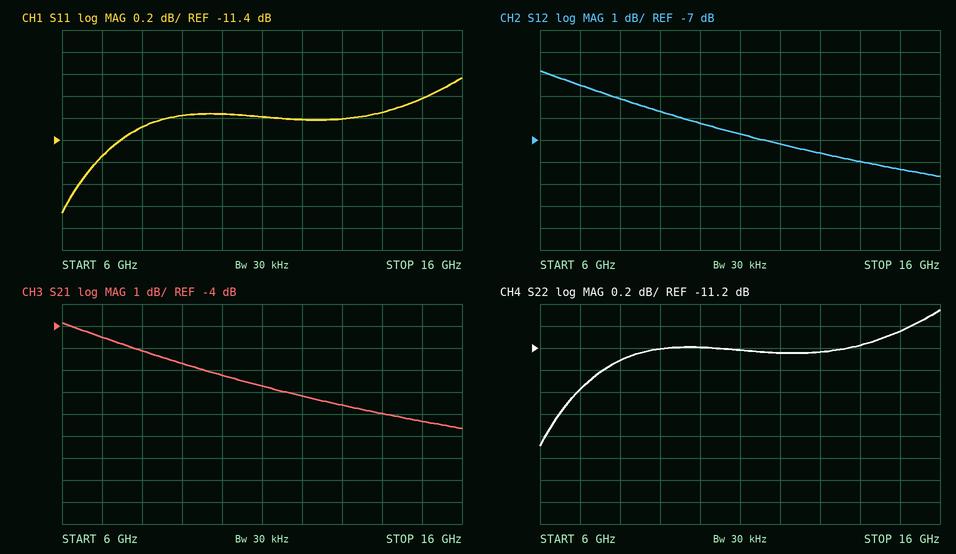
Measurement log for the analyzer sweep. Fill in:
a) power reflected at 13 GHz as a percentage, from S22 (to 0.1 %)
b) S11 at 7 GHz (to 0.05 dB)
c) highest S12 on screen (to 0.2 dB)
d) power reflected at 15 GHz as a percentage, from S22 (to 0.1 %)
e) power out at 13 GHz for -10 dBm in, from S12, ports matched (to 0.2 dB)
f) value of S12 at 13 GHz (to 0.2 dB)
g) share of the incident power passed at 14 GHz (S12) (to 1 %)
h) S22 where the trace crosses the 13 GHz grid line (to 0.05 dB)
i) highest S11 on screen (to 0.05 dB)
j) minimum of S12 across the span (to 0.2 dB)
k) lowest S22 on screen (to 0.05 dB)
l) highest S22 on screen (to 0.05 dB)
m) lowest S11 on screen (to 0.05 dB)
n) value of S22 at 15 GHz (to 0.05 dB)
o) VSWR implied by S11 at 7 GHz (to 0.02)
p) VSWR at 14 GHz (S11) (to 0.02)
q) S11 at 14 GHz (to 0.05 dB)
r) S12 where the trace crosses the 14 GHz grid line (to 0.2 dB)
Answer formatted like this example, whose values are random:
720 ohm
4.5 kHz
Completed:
7.5 %
-11.55 dB
-3.8 dB
7.9 %
-17.6 dBm
-7.6 dB
16 %
-11.25 dB
-10.85 dB
-8.6 dB
-12.10 dB
-10.85 dB
-12.05 dB
-11.05 dB
1.72
1.76
-11.15 dB
-8.0 dB
